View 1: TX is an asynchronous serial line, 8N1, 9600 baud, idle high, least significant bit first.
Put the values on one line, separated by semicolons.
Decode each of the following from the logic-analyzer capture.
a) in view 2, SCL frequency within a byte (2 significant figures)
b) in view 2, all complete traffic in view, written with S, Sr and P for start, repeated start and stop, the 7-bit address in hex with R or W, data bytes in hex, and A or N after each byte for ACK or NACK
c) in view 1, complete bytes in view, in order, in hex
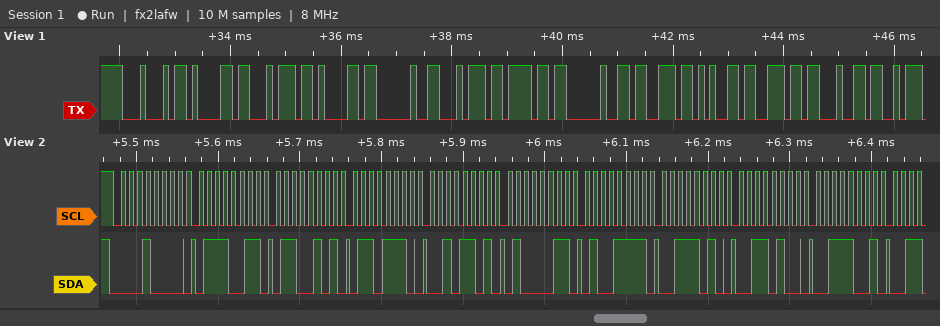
100 kHz; S 08W A 73 A 65 A 6E A 2D A 43 A 4F A 3A A 34 A 39 A; 44 61 74 61 20 74 6F 20 73 65 6E 64
